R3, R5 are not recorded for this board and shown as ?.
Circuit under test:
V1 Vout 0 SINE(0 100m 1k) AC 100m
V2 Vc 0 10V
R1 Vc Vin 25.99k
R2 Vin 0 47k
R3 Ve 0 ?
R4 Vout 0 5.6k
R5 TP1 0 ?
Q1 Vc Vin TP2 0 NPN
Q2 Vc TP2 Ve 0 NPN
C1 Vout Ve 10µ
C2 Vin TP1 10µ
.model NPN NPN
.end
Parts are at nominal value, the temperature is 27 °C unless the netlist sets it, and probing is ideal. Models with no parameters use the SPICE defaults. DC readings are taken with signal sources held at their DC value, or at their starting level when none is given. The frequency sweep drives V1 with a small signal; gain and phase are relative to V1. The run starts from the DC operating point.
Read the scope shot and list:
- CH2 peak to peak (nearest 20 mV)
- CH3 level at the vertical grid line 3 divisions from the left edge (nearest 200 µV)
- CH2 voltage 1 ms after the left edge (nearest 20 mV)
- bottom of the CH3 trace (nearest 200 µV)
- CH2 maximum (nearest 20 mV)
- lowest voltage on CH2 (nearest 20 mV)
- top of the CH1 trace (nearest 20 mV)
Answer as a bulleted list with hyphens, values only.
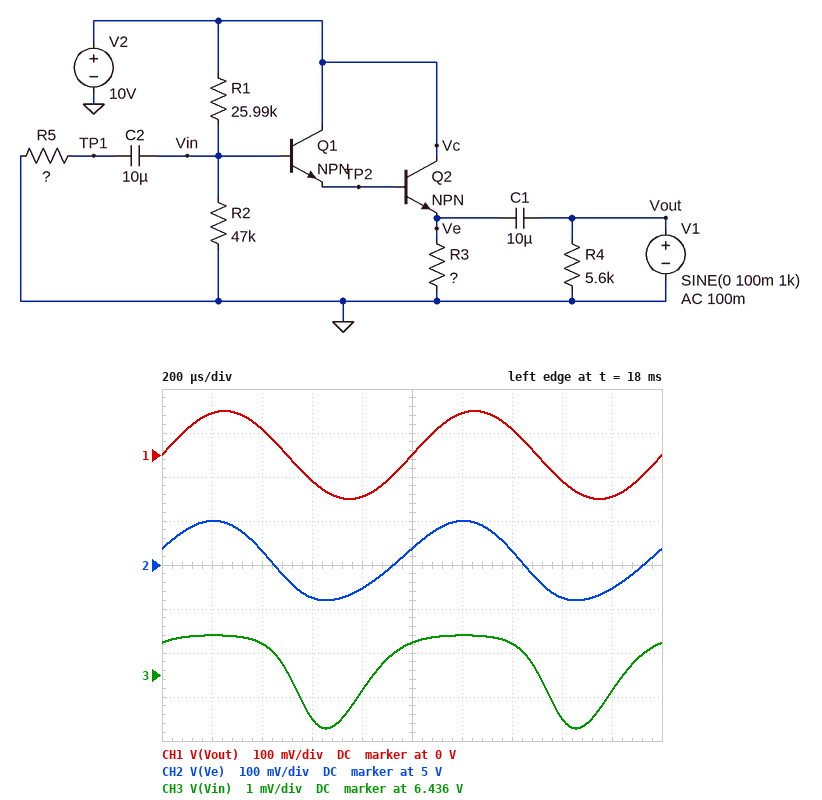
- 180 mV
- 6.4350 V
- 5.04 V
- 6.4348 V
- 5.10 V
- 4.92 V
- 100 mV
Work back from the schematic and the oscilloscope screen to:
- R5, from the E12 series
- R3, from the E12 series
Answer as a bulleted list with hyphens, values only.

- 5.6 kΩ
- 2.7 kΩ
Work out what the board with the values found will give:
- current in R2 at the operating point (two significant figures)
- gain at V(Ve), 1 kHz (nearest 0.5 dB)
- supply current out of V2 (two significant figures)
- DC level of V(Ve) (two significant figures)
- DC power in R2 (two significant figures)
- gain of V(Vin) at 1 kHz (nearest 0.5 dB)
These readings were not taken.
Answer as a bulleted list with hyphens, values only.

- 140 µA
- -1.0 dB
- 2.0 mA
- 5.0 V
- 880 µW
- -38.0 dB
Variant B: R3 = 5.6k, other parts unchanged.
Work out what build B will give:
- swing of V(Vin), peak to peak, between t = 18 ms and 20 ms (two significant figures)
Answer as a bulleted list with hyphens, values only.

- 1.1 mV
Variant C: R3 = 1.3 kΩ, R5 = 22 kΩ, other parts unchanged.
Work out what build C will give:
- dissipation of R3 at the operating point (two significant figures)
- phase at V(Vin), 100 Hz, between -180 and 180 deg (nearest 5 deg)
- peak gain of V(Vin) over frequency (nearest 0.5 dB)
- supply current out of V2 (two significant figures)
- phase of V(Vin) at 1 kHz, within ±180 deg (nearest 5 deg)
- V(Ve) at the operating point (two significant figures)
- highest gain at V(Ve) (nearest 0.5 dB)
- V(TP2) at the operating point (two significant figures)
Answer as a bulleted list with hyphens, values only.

- 19 mW
- 85 deg
- -24.0 dB
- 3.9 mA
- 50 deg
- 4.9 V
- 0 dB
- 5.7 V
